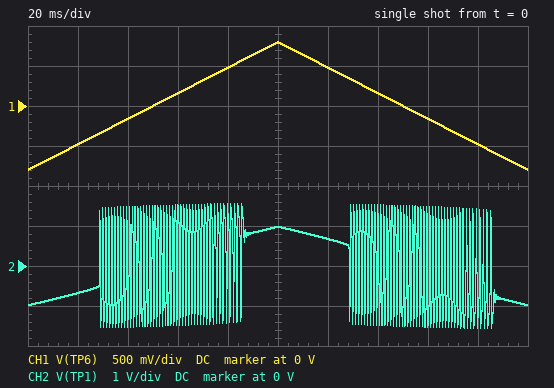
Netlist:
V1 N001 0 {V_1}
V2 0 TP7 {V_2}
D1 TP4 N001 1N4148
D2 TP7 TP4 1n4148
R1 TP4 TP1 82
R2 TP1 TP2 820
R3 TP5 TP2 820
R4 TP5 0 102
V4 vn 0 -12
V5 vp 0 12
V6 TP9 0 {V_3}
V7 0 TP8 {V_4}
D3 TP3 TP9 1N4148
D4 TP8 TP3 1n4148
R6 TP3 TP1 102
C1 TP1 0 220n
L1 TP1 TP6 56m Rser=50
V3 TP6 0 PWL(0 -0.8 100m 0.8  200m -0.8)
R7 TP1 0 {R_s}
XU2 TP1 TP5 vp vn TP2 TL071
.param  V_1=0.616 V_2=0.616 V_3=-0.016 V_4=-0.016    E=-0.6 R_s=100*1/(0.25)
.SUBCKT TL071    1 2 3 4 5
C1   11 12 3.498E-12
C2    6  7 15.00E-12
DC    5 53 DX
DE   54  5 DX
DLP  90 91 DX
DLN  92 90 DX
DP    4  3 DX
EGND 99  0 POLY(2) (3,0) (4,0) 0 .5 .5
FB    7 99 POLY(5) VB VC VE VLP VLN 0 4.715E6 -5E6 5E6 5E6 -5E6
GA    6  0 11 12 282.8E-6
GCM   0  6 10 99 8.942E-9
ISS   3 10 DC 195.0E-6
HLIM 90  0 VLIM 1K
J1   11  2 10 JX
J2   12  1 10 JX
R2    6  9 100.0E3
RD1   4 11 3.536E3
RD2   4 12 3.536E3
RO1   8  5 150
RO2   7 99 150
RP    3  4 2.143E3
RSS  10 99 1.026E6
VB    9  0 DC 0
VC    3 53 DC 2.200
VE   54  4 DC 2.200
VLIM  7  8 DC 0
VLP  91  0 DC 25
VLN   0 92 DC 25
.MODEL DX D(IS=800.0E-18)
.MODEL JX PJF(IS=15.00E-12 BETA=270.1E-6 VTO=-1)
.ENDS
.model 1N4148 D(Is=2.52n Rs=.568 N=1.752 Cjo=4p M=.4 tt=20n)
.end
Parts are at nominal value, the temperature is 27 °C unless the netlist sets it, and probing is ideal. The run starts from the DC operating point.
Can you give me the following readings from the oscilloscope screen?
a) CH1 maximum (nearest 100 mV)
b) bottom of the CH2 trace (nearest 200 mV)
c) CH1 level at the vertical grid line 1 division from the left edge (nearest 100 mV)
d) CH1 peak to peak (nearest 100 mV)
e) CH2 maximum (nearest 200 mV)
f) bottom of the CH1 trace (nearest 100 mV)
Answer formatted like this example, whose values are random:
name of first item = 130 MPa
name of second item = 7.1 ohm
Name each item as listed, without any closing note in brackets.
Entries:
CH1 maximum = 800 mV
bottom of the CH2 trace = -1.6 V
CH1 level at the vertical grid line 1 division from the left edge = -500 mV
CH1 peak to peak = 1.6 V
CH2 maximum = 1.6 V
bottom of the CH1 trace = -800 mV
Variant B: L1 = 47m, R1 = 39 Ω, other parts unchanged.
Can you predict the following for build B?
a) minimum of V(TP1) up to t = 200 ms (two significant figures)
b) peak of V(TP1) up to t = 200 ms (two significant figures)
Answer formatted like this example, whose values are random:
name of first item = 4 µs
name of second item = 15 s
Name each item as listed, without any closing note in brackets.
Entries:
minimum of V(TP1) up to t = 200 ms = -1.5 V
peak of V(TP1) up to t = 200 ms = 1.5 V
